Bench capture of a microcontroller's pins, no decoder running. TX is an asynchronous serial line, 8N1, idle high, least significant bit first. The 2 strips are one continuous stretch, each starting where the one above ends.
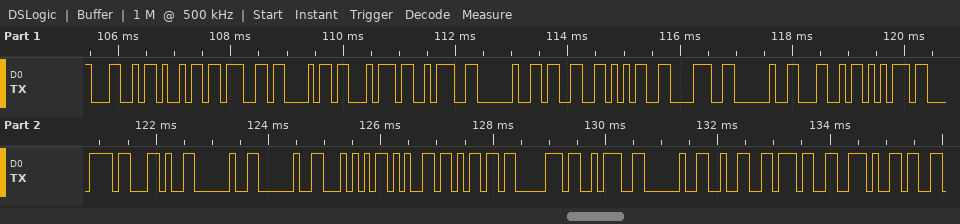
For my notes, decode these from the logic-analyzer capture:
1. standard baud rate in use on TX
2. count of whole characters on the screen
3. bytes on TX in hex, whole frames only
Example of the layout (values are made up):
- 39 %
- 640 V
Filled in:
- 9600 baud
- 26
- 4C 69 67 68 74 3A 20 33 35 38 20 4C 75 78 2C 20 20 54 65 6D 70 3A 20 32 37 2E
